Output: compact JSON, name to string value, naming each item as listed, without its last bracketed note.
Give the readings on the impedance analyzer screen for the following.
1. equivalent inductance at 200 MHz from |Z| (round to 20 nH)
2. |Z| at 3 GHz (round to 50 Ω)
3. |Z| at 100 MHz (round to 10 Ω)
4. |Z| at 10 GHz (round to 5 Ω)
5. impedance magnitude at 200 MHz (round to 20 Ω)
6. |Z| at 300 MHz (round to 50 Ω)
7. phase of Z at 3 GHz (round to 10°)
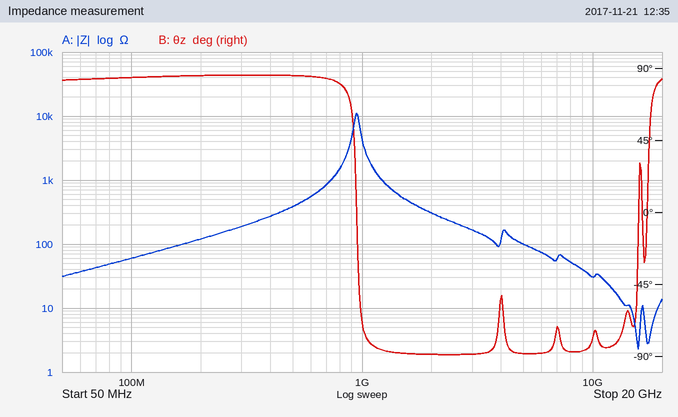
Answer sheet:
{"equivalent inductance at 200 MHz from |Z|": "100 nH", "|Z| at 3 GHz": "150 Ω", "|Z| at 100 MHz": "60 Ω", "|Z| at 10 GHz": "30 Ω", "impedance magnitude at 200 MHz": "120 Ω", "|Z| at 300 MHz": "200 Ω", "phase of Z at 3 GHz": "-90°"}
